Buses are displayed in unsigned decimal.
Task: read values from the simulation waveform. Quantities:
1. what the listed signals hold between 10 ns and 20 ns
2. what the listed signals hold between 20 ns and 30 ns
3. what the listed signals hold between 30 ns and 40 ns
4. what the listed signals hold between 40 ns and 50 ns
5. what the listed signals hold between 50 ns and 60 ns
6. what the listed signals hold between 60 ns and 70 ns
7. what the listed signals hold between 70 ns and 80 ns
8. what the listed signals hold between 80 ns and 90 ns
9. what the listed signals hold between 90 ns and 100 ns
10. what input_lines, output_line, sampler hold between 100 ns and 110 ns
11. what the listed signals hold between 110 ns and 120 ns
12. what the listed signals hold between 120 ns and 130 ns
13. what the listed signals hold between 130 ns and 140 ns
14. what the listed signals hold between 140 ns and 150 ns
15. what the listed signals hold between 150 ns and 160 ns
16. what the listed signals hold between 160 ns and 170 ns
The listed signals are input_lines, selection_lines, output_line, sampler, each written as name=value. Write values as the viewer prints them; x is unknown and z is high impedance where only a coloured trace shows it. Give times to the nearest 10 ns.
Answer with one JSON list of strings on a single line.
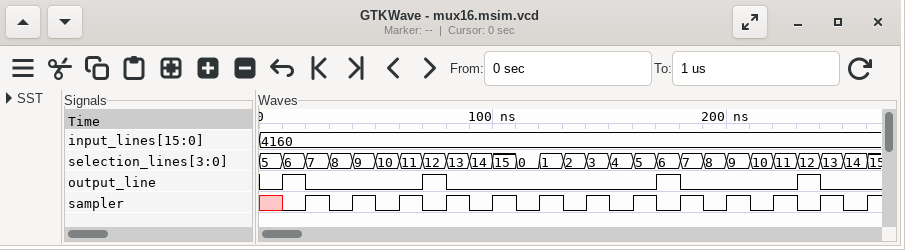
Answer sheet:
["input_lines=4160, selection_lines=6, output_line=1, sampler=0", "input_lines=4160, selection_lines=7, output_line=0, sampler=1", "input_lines=4160, selection_lines=8, output_line=0, sampler=0", "input_lines=4160, selection_lines=9, output_line=0, sampler=1", "input_lines=4160, selection_lines=10, output_line=0, sampler=0", "input_lines=4160, selection_lines=11, output_line=0, sampler=1", "input_lines=4160, selection_lines=12, output_line=1, sampler=0", "input_lines=4160, selection_lines=13, output_line=0, sampler=1", "input_lines=4160, selection_lines=14, output_line=0, sampler=0", "input_lines=4160, output_line=0, sampler=1", "input_lines=4160, selection_lines=0, output_line=0, sampler=0", "input_lines=4160, selection_lines=1, output_line=0, sampler=1", "input_lines=4160, selection_lines=2, output_line=0, sampler=0", "input_lines=4160, selection_lines=3, output_line=0, sampler=1", "input_lines=4160, selection_lines=4, output_line=0, sampler=0", "input_lines=4160, selection_lines=5, output_line=0, sampler=1"]
